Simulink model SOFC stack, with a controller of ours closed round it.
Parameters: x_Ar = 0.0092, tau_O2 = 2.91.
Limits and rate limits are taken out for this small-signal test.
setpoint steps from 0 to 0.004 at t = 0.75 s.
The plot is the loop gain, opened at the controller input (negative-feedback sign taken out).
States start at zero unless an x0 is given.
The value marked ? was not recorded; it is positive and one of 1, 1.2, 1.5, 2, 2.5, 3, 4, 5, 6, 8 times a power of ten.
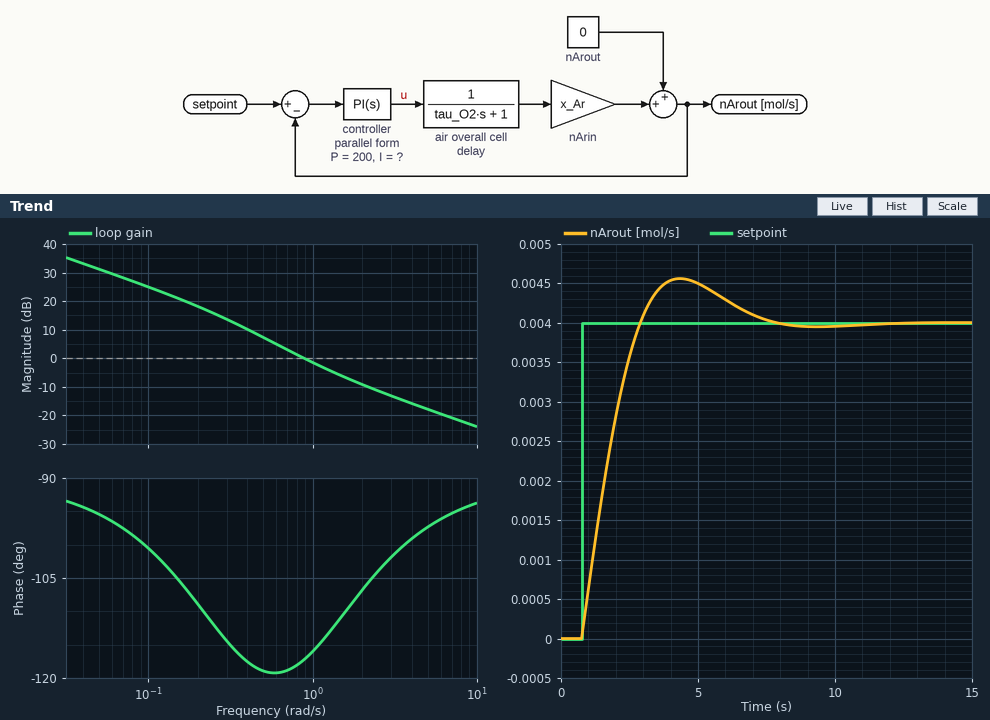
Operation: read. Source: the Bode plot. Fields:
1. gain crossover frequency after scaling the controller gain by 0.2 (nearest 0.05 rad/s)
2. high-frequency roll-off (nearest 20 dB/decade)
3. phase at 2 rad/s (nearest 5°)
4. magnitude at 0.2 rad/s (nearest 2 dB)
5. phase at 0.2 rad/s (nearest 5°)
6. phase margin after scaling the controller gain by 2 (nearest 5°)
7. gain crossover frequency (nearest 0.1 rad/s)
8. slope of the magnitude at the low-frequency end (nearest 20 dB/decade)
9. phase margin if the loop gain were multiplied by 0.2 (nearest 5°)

0.30 rad/s
-20 dB/decade
-105°
18 dB
-110°
70°
0.9 rad/s
-20 dB/decade
65°
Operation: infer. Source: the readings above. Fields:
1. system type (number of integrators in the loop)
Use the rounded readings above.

1
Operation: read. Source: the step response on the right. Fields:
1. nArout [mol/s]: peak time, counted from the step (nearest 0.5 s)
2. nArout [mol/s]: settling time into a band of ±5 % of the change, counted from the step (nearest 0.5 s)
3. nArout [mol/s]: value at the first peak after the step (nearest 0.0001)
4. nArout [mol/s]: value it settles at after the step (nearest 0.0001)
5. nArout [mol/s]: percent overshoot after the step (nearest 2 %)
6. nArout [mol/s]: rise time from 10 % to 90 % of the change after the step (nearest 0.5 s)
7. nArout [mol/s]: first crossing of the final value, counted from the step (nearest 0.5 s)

3.5 s
5.5 s
0.0046
0.0040
14 %
1.5 s
2.0 s
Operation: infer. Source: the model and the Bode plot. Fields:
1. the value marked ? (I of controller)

200
